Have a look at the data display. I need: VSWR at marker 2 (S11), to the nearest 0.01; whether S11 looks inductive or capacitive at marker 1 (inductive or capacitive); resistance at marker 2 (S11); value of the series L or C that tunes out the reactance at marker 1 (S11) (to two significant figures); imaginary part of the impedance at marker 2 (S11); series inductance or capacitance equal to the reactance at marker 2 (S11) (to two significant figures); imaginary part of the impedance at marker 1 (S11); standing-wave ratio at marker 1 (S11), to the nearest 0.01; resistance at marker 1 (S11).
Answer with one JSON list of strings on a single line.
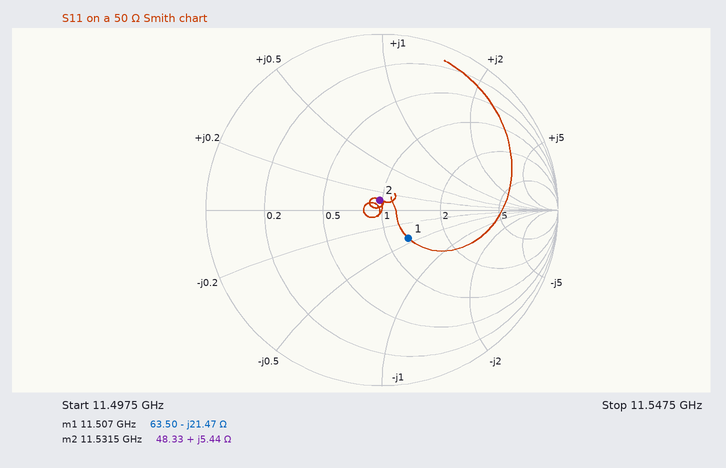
["1.12", "capacitive", "48.33 Ω", "300 pH", "+5.44 Ω", "75 pH", "-21.47 Ω", "1.56", "63.50 Ω"]
